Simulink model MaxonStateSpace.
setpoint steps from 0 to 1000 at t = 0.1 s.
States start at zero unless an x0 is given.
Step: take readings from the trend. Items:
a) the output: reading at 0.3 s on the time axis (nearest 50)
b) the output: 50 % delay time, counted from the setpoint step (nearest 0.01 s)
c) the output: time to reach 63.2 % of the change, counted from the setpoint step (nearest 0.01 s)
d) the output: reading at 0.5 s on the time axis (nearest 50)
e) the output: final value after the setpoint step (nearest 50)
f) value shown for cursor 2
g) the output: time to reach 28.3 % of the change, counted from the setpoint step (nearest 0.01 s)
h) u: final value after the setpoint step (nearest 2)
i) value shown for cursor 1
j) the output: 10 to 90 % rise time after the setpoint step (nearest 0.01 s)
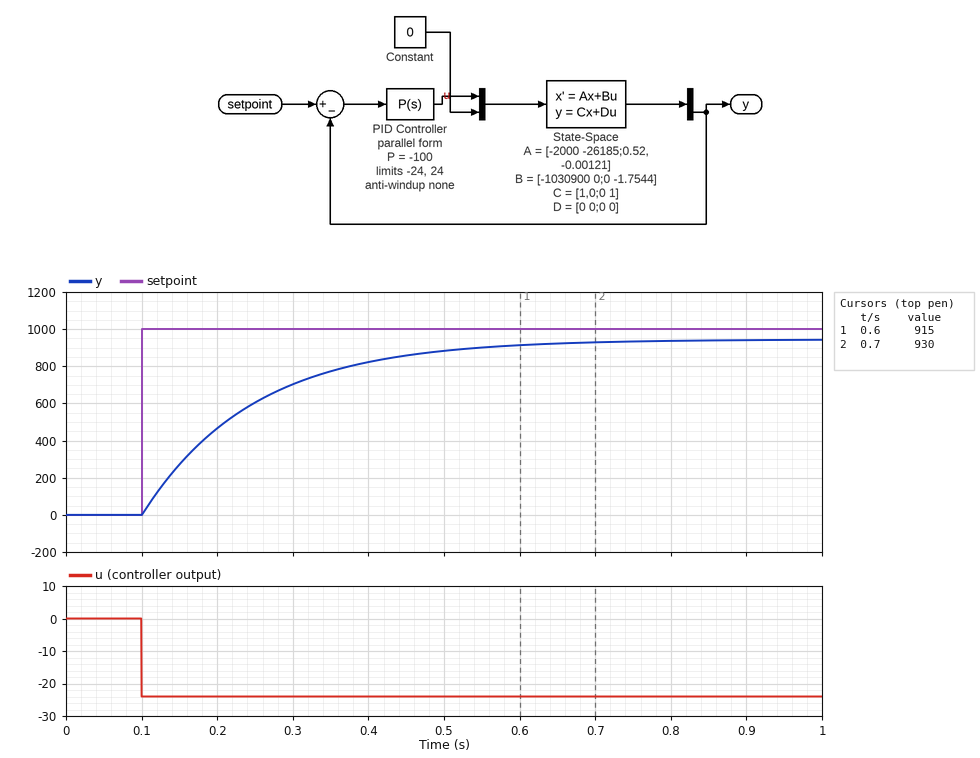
700
0.10 s
0.15 s
900
950
930
0.05 s
-24
915
0.32 s
